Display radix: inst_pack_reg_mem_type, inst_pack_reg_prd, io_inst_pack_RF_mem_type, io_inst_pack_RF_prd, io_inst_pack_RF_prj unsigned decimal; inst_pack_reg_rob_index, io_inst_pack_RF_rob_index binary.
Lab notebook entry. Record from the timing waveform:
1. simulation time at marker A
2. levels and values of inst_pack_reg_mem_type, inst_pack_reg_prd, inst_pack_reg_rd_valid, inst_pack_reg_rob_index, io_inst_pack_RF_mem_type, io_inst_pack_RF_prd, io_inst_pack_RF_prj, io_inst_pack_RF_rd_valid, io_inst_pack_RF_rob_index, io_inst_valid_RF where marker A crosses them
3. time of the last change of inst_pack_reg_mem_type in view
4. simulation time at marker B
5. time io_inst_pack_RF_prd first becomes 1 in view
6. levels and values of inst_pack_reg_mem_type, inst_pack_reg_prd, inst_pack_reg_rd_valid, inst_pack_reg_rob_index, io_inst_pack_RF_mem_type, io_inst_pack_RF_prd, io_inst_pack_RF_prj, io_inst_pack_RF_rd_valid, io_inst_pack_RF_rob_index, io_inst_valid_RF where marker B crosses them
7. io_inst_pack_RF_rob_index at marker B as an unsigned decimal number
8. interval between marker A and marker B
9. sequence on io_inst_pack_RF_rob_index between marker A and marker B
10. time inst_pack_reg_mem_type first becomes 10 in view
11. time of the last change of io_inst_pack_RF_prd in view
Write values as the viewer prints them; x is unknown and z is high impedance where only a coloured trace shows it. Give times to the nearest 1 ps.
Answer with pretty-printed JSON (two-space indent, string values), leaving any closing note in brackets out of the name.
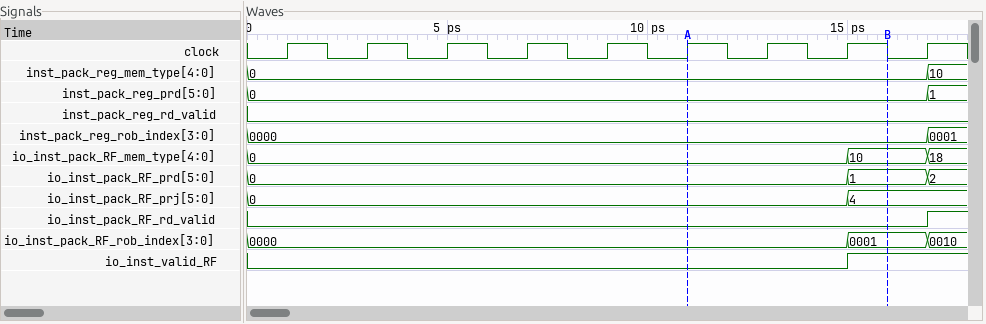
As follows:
{
  "simulation time at marker A": "11 ps",
  "levels and values of inst_pack_reg_mem_type, inst_pack_reg_prd, inst_pack_reg_rd_valid, inst_pack_reg_rob_index, io_inst_pack_RF_mem_type, io_inst_pack_RF_prd, io_inst_pack_RF_prj, io_inst_pack_RF_rd_valid, io_inst_pack_RF_rob_index, io_inst_valid_RF where marker A crosses them": "inst_pack_reg_mem_type=0, inst_pack_reg_prd=0, inst_pack_reg_rd_valid=0, inst_pack_reg_rob_index=0000, io_inst_pack_RF_mem_type=0, io_inst_pack_RF_prd=0, io_inst_pack_RF_prj=0, io_inst_pack_RF_rd_valid=0, io_inst_pack_RF_rob_index=0000, io_inst_valid_RF=0",
  "time of the last change of inst_pack_reg_mem_type in view": "17 ps",
  "simulation time at marker B": "16 ps",
  "time io_inst_pack_RF_prd first becomes 1 in view": "15 ps",
  "levels and values of inst_pack_reg_mem_type, inst_pack_reg_prd, inst_pack_reg_rd_valid, inst_pack_reg_rob_index, io_inst_pack_RF_mem_type, io_inst_pack_RF_prd, io_inst_pack_RF_prj, io_inst_pack_RF_rd_valid, io_inst_pack_RF_rob_index, io_inst_valid_RF where marker B crosses them": "inst_pack_reg_mem_type=0, inst_pack_reg_prd=0, inst_pack_reg_rd_valid=0, inst_pack_reg_rob_index=0000, io_inst_pack_RF_mem_type=10, io_inst_pack_RF_prd=1, io_inst_pack_RF_prj=4, io_inst_pack_RF_rd_valid=0, io_inst_pack_RF_rob_index=0001, io_inst_valid_RF=1",
  "io_inst_pack_RF_rob_index at marker B as an unsigned decimal number": "1",
  "interval between marker A and marker B": "5 ps",
  "sequence on io_inst_pack_RF_rob_index between marker A and marker B": "0000, 0001",
  "time inst_pack_reg_mem_type first becomes 10 in view": "17 ps",
  "time of the last change of io_inst_pack_RF_prd in view": "17 ps"
}
